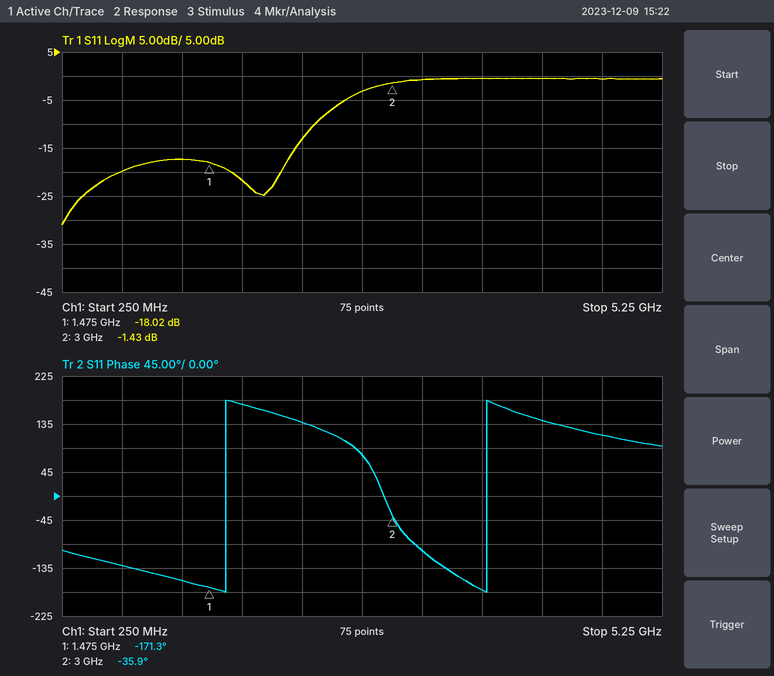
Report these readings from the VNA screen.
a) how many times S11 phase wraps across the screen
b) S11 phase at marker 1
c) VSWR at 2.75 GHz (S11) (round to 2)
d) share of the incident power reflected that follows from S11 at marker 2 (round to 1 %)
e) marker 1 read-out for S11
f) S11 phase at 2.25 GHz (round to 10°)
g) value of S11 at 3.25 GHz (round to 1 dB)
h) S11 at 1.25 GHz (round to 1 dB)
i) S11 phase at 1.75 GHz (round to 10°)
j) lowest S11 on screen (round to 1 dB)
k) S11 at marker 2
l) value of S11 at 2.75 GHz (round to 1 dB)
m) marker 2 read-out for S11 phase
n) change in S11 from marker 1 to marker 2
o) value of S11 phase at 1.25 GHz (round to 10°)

2
-171.3°
6
72 %
-18.02 dB
140°
-1 dB
-17 dB
170°
-31 dB
-1.43 dB
-3 dB
-35.9°
16.59 dB
-160°
